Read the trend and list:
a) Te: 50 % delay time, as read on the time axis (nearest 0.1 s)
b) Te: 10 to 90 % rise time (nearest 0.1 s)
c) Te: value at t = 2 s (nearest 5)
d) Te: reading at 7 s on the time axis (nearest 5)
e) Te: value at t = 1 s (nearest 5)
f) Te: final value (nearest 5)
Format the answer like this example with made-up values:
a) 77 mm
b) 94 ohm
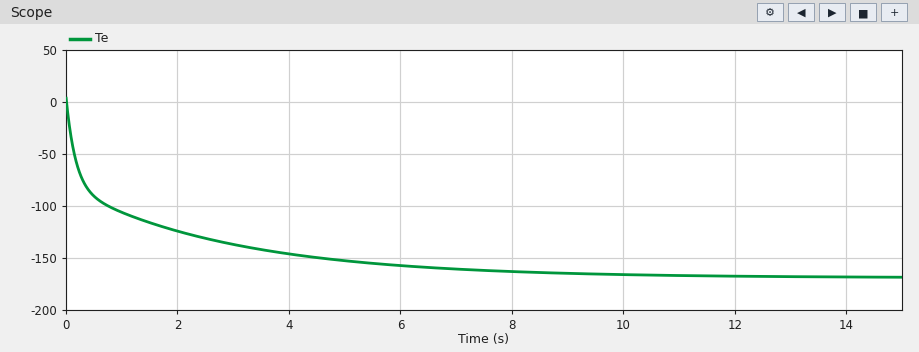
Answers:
a) 0.4 s
b) 4.8 s
c) -125
d) -160
e) -105
f) -170
